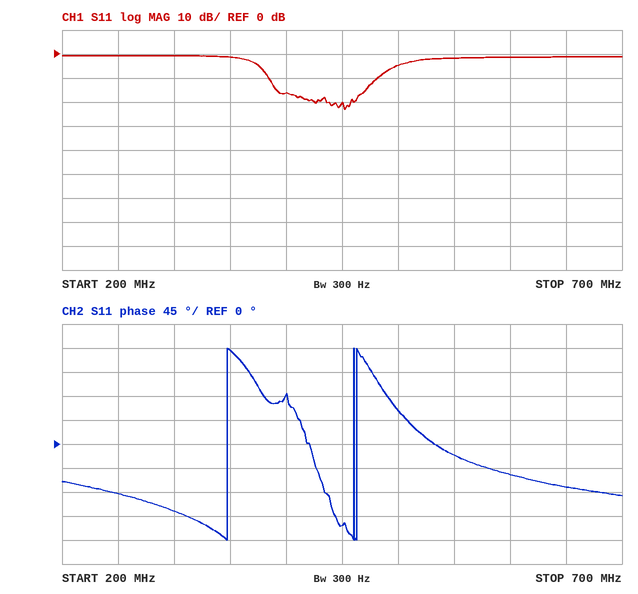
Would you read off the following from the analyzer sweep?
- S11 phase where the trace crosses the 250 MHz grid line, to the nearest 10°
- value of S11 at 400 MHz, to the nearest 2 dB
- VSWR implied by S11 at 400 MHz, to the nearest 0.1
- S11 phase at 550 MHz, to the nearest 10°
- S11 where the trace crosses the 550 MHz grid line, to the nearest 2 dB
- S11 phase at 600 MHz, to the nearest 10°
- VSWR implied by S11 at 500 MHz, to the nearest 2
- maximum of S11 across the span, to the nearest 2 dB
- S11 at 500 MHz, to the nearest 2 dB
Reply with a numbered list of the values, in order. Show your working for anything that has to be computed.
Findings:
1. -90°
2. -16 dB
3. |Γ| = 10^(-16/20) = 0.1585; VSWR = (1 + 0.1585)/(1 − 0.1585) ≈ 1.4
4. -20°
5. -2 dB
6. -60°
7. |Γ| = 10^(-4/20) = 0.6310; VSWR = (1 + 0.6310)/(1 − 0.6310) ≈ 4
8. 0 dB
9. -4 dB
